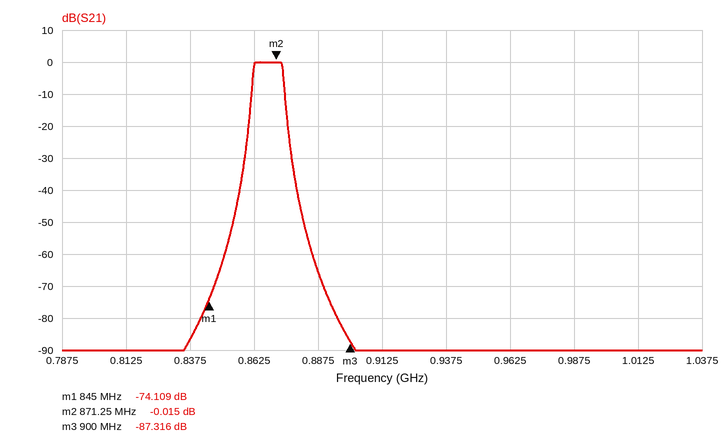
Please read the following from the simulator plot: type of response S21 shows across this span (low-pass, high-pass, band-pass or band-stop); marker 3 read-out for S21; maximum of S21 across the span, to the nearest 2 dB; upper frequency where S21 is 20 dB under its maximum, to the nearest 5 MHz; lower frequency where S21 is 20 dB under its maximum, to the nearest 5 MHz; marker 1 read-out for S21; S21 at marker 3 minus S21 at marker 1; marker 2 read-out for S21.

band-pass
-87.316 dB
0 dB
875 MHz
860 MHz
-74.109 dB
-13.207 dB
-0.015 dB
